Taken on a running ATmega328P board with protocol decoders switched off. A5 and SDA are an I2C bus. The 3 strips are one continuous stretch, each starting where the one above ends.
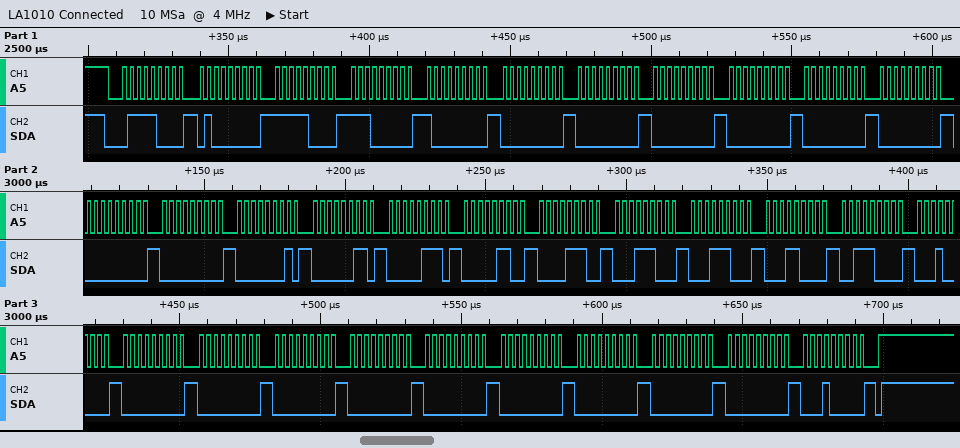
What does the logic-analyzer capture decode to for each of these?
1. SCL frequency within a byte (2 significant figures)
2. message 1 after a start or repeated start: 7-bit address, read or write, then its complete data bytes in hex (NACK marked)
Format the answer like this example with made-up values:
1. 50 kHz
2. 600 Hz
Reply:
1. 400 kHz
2. 0x3C write: 40 F8 E0 80 00 00 00 00 00 00 00 00 01 03 07 06 0E 1C 1C 18 38 10 00 00 00 00 00 00 00 00 00 10
